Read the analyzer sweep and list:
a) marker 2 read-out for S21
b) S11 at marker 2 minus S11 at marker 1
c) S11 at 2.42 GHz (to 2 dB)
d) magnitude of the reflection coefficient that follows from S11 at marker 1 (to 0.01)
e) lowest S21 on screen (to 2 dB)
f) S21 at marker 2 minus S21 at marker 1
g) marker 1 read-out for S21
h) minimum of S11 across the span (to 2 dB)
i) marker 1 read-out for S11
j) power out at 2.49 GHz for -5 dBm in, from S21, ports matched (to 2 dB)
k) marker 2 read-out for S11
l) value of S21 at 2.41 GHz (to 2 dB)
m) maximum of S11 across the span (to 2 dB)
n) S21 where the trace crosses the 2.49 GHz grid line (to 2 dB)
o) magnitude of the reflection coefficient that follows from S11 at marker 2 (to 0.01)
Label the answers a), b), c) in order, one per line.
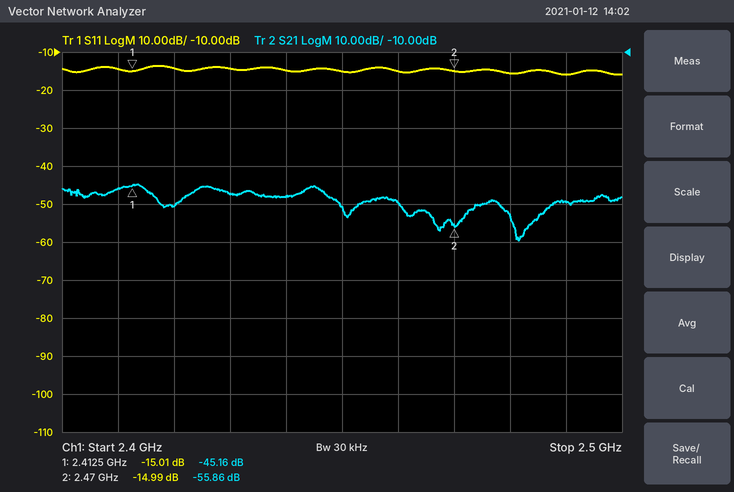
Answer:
a) -55.86 dB
b) 0.02 dB
c) -14 dB
d) 0.18
e) -60 dB
f) -10.70 dB
g) -45.16 dB
h) -16 dB
i) -15.01 dB
j) -54 dBm
k) -14.99 dB
l) -46 dB
m) -14 dB
n) -50 dB
o) 0.18
